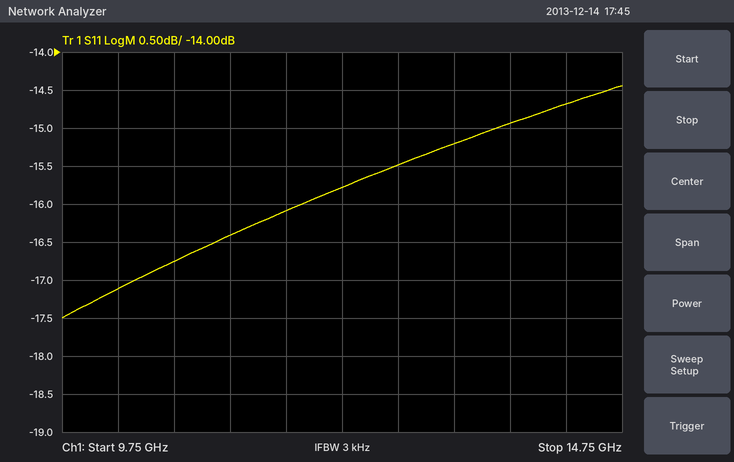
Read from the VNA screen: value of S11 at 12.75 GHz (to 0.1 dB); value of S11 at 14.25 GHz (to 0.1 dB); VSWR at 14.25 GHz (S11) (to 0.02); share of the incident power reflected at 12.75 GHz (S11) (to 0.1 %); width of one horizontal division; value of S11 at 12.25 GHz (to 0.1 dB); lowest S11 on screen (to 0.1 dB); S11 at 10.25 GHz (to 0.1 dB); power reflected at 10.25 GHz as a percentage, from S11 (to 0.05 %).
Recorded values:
-15.5 dB
-14.7 dB
1.46
2.8 %
500 MHz
-15.8 dB
-17.5 dB
-17.1 dB
1.95 %
